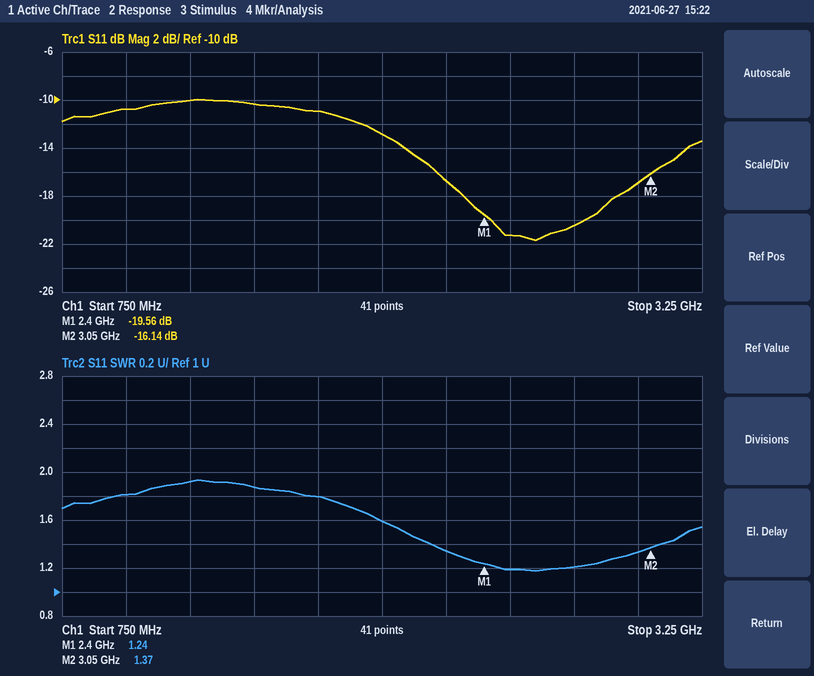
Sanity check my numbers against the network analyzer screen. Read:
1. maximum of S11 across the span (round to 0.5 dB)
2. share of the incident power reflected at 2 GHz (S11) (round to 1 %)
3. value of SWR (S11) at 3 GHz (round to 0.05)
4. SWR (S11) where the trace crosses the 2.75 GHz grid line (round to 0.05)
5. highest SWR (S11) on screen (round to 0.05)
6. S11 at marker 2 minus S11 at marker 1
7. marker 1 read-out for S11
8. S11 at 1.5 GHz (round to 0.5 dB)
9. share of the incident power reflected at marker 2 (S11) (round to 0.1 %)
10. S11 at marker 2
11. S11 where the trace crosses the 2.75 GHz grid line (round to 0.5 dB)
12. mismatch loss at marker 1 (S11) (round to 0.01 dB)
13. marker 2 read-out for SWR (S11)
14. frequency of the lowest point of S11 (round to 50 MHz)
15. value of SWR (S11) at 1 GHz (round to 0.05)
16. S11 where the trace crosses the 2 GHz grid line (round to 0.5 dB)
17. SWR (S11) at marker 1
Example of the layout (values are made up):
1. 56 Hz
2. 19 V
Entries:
1. -10.0 dB
2. 5 %
3. 1.35
4. 1.20
5. 1.95
6. 3.42 dB
7. -19.56 dB
8. -10.5 dB
9. 2.4 %
10. -16.14 dB
11. -20.5 dB
12. 0.05 dB
13. 1.37
14. 2.60 GHz
15. 1.80
16. -13.0 dB
17. 1.24
